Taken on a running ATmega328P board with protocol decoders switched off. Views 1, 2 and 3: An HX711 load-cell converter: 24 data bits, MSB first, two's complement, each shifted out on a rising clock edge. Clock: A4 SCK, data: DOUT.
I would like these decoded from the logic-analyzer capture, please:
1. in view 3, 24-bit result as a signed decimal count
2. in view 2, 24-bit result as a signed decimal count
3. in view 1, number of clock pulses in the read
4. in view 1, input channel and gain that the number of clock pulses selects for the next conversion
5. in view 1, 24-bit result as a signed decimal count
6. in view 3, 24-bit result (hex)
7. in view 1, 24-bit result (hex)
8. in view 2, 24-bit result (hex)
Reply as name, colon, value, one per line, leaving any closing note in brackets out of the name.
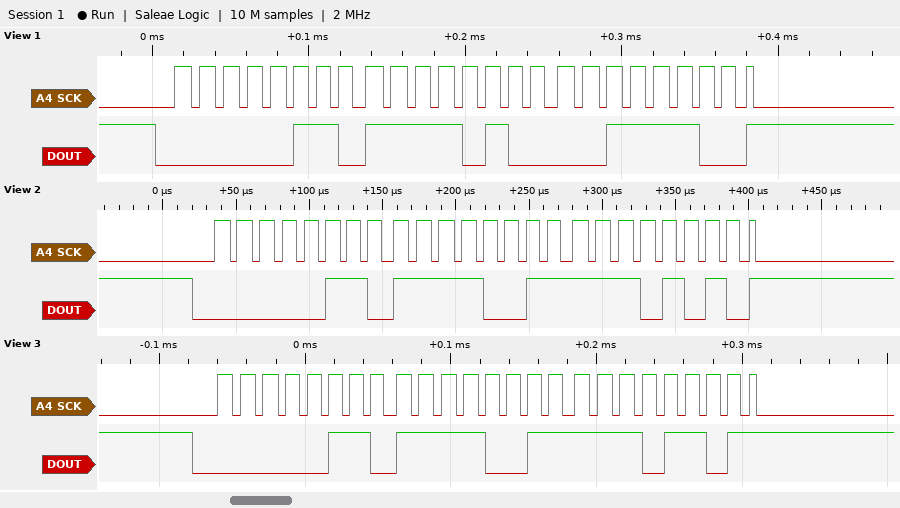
in view 3, 24-bit result as a signed decimal count: 455661
in view 2, 24-bit result as a signed decimal count: 455658
in view 1, number of clock pulses in the read: 25
in view 1, input channel and gain that the number of clock pulses selects for the next conversion: channel A, gain 128
in view 1, 24-bit result as a signed decimal count: 455740
in view 3, 24-bit result: 0x06F3ED
in view 1, 24-bit result: 0x06F43C
in view 2, 24-bit result: 0x06F3EA
